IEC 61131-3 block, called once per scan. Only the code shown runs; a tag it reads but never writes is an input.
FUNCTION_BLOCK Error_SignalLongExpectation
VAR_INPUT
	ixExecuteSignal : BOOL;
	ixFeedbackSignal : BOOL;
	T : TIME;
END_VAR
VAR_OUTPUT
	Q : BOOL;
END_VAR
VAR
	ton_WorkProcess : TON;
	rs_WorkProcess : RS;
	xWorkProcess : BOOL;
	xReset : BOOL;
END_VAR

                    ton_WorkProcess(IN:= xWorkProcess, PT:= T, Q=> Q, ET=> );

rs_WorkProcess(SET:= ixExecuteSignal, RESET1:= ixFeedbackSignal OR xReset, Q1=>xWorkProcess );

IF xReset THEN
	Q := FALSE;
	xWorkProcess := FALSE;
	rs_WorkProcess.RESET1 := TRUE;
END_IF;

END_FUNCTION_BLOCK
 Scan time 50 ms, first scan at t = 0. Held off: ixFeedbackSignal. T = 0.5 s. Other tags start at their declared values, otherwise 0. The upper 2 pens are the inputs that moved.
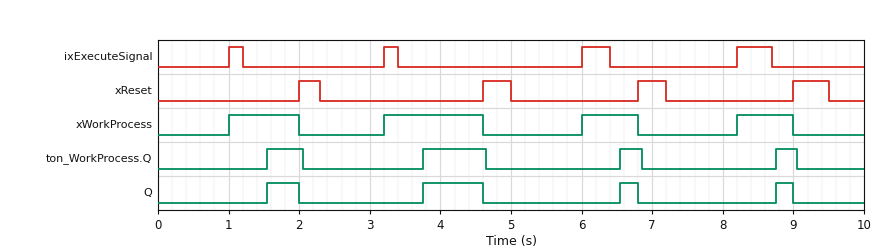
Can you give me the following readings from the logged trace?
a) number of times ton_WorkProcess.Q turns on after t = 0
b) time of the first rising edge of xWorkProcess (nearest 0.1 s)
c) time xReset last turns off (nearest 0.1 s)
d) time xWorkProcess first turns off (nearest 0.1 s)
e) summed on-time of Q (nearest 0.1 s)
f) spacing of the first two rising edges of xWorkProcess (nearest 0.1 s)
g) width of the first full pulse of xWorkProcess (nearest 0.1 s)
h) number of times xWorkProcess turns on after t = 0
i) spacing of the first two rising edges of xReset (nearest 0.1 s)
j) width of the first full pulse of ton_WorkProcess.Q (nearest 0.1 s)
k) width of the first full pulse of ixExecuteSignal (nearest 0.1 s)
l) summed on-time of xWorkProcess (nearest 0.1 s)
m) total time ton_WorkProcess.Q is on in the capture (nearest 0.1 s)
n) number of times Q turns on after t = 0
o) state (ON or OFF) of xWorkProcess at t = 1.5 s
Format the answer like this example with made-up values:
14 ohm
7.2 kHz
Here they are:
4
1.0 s
9.5 s
2.0 s
1.8 s
2.2 s
1.0 s
4
2.6 s
0.5 s
0.2 s
4.0 s
2.0 s
4
ON
